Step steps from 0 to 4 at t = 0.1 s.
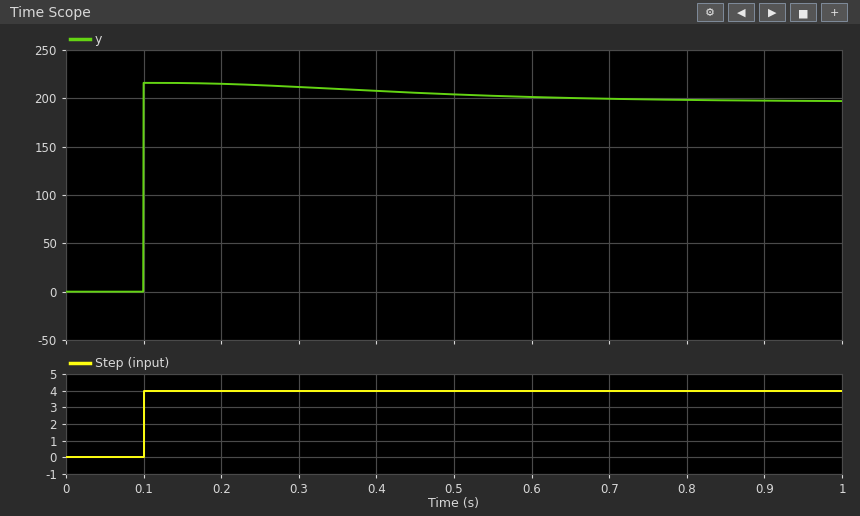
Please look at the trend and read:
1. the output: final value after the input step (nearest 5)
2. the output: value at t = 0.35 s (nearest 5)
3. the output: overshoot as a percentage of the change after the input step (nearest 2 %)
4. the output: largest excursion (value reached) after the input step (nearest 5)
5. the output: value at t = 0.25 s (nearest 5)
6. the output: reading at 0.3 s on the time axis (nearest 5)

195
210
10 %
215
215
210
